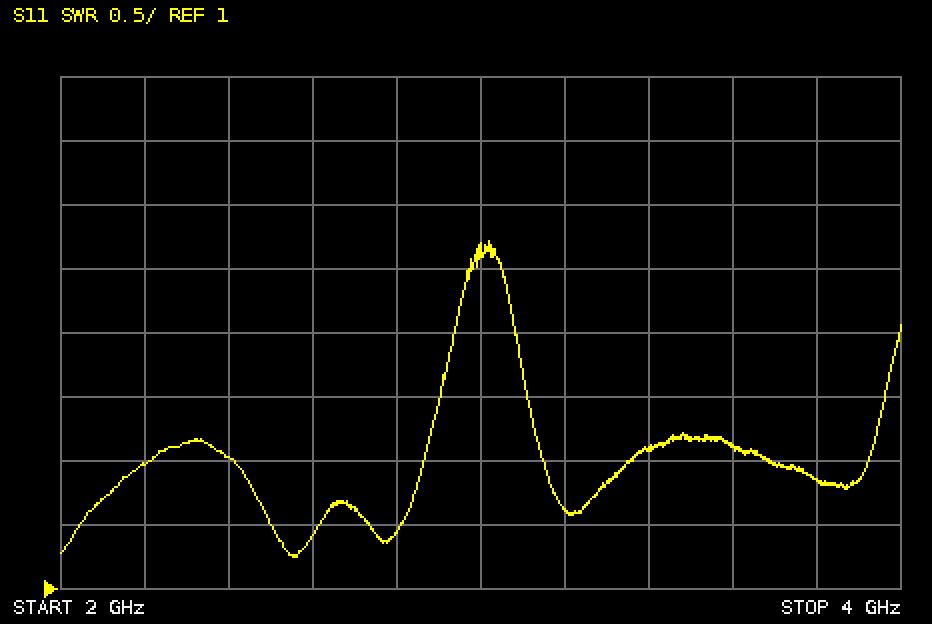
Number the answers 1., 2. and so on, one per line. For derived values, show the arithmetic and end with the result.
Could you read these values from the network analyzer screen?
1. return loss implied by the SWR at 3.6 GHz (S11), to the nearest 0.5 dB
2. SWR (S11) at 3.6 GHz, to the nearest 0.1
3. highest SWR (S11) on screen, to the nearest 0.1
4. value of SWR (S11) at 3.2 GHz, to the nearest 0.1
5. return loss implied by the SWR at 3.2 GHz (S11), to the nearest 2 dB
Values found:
1. −20 log10((2.1 − 1)/(2.1 + 1)) ≈ 9.0 dB
2. 2.1
3. 3.7
4. 1.6
5. −20 log10((1.6 − 1)/(1.6 + 1)) ≈ 12.7 dB, so 12 dB to the nearest 2 dB
